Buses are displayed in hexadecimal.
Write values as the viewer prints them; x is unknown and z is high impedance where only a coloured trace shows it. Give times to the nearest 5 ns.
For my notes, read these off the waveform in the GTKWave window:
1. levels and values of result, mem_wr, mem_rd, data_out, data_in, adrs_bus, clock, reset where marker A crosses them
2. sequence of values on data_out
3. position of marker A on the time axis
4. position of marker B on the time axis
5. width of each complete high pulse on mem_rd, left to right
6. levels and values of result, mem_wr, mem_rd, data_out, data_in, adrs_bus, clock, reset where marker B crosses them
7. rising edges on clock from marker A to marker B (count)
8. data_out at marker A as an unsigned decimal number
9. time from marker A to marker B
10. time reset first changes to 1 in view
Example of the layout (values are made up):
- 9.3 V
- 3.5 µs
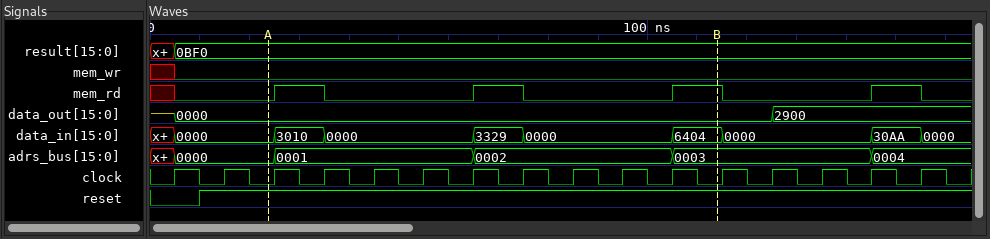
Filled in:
- result=0BF0, mem_wr=0, mem_rd=0, data_out=0000, data_in=0000, adrs_bus=0000, clock=0, reset=1
- z, 0000, 2900
- 25 ns
- 115 ns
- 10 ns, 10 ns, 10 ns, 10 ns
- result=0BF0, mem_wr=0, mem_rd=1, data_out=0000, data_in=6404, adrs_bus=0003, clock=0, reset=1
- 9
- 0
- 90 ns
- 10 ns
